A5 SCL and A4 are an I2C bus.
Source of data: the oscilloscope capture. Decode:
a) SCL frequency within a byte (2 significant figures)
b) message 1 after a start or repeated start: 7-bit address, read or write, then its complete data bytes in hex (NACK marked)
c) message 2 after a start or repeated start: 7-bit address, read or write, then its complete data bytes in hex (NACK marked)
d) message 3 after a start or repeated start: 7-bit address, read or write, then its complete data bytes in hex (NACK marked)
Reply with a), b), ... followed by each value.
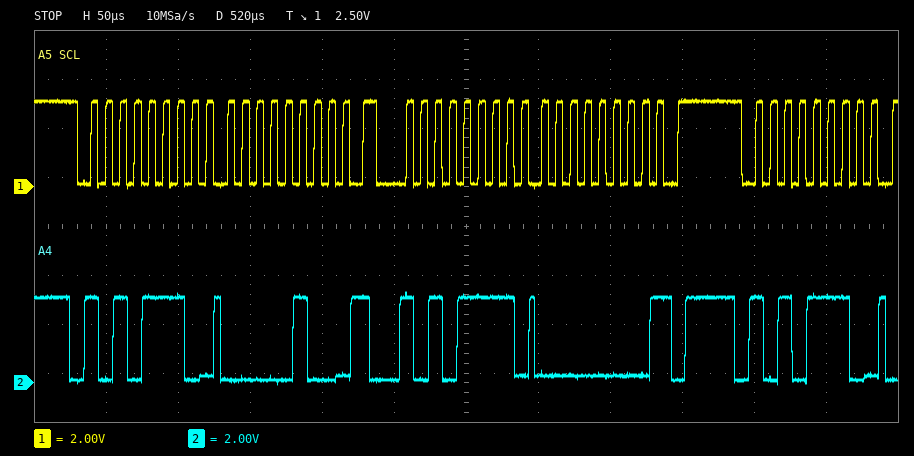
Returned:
a) 100 kHz
b) 0x57 write: 04
c) 0x57 read: 00 NACK
d) 0x57 write
